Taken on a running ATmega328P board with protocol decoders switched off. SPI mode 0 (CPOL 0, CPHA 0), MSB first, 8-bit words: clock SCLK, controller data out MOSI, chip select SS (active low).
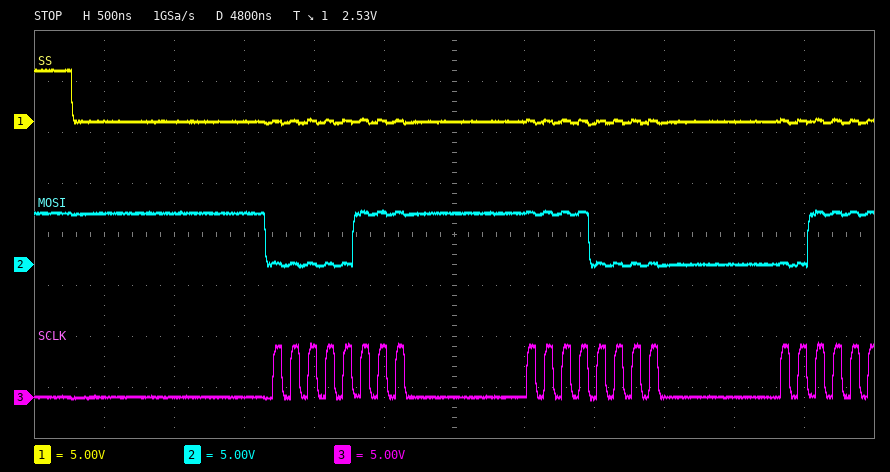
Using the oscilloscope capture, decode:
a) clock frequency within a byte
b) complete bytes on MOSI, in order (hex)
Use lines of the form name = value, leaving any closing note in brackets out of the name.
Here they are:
clock frequency within a byte = 8 MHz
complete bytes on MOSI, in order = 07 F0
